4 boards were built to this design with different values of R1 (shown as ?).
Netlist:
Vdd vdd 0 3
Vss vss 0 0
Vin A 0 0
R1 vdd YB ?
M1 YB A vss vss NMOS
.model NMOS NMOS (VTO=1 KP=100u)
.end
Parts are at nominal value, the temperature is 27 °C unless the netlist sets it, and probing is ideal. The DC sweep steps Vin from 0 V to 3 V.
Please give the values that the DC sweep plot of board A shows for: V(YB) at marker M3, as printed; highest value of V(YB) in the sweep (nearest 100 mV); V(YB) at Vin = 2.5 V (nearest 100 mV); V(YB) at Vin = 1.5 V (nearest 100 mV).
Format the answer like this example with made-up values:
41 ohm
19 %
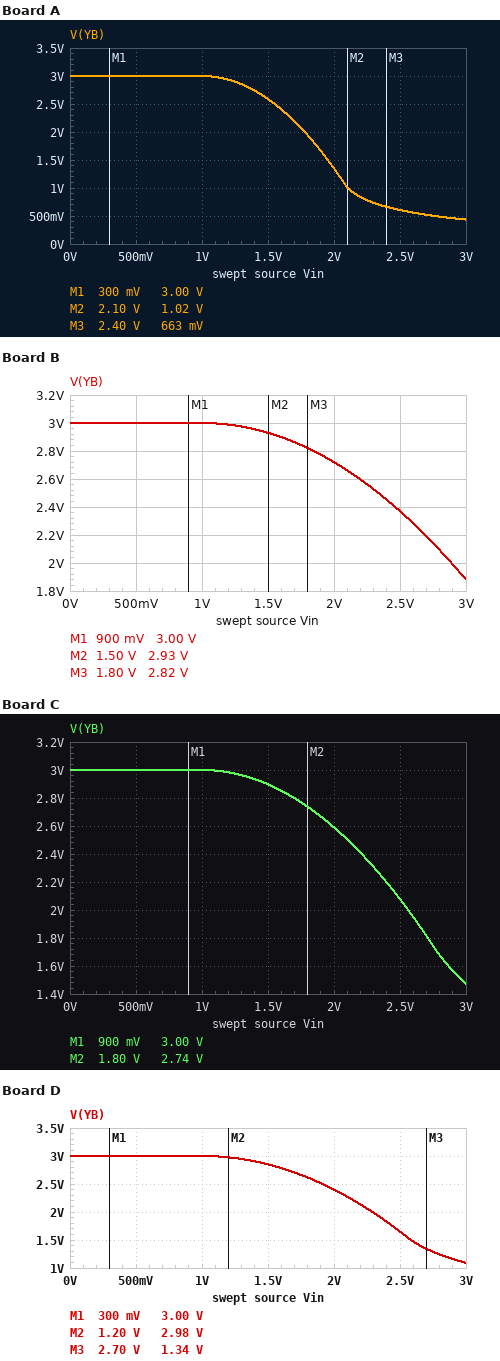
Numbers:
663 mV
3.0 V
600 mV
2.6 V
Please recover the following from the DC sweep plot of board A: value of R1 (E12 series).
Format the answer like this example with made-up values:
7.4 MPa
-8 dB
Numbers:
33 kΩ
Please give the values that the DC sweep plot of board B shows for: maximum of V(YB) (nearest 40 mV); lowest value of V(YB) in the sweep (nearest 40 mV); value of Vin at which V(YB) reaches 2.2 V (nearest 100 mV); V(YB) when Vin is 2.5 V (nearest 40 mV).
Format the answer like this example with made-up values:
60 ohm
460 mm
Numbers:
3.00 V
1.88 V
2.7 V
2.36 V
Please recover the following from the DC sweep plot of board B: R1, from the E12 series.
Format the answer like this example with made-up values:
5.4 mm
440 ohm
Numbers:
5.6 kΩ
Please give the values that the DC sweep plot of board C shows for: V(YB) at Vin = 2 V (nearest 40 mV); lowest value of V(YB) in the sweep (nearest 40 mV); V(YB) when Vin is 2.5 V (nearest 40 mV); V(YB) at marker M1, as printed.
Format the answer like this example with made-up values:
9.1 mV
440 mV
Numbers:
2.60 V
1.48 V
2.08 V
3.00 V
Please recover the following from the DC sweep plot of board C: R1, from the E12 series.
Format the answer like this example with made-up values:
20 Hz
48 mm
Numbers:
8.2 kΩ
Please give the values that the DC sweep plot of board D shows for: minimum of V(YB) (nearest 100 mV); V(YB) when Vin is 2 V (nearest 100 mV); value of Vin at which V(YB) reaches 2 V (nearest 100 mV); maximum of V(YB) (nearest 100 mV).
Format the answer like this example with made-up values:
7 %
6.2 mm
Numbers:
1.1 V
2.4 V
2.3 V
3.0 V
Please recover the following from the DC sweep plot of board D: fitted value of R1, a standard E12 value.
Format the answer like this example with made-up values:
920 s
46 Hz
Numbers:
12 kΩ
